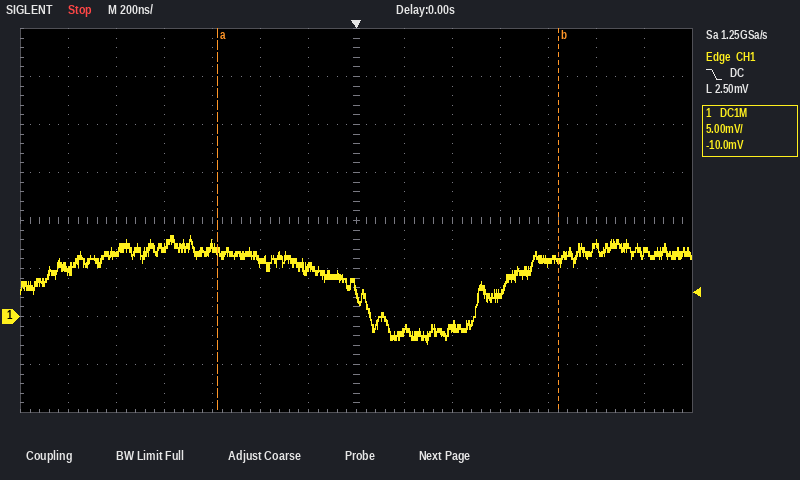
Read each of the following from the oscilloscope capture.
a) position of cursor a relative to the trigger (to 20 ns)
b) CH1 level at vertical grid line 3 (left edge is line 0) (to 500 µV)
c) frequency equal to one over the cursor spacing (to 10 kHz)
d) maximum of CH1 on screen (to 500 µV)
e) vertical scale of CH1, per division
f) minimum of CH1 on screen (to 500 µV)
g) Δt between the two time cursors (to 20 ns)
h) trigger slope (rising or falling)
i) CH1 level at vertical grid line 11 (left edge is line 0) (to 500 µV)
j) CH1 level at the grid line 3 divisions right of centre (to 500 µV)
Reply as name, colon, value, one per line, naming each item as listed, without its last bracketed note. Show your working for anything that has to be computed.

position of cursor a relative to the trigger: -580 ns
CH1 level at vertical grid line 3 (left edge is line 0): 7.0 mV
frequency equal to one over the cursor spacing: 1 / 1.42 µs ≈ 700 kHz
maximum of CH1 on screen: 8.5 mV
vertical scale of CH1, per division: 5 mV
minimum of CH1 on screen: -3.0 mV
Δt between the two time cursors: 1.42 µs
trigger slope: falling
CH1 level at vertical grid line 11 (left edge is line 0): 5.5 mV
CH1 level at the grid line 3 divisions right of centre: 2.5 mV
